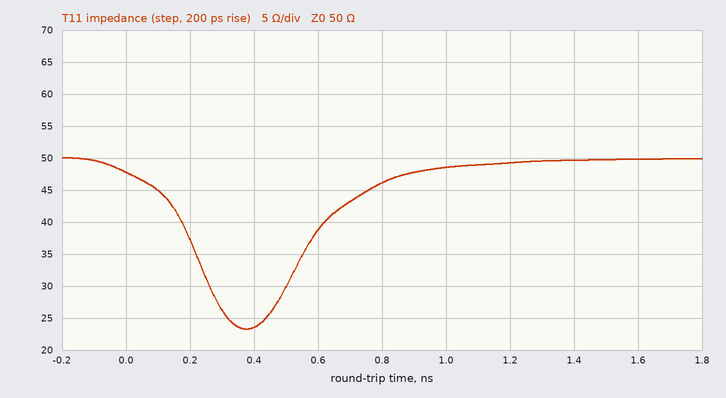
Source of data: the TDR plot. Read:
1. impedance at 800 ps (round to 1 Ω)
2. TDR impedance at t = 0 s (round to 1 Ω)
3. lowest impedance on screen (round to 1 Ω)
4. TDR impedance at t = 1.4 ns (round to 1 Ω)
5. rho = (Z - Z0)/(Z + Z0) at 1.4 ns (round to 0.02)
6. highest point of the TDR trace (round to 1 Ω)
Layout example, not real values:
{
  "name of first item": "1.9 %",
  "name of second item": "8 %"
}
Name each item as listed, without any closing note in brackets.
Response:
{
  "impedance at 800 ps": "46 Ω",
  "TDR impedance at t = 0 s": "48 Ω",
  "lowest impedance on screen": "23 Ω",
  "TDR impedance at t = 1.4 ns": "50 Ω",
  "rho = (Z - Z0)/(Z + Z0) at 1.4 ns": "0.00",
  "highest point of the TDR trace": "50 Ω"
}
